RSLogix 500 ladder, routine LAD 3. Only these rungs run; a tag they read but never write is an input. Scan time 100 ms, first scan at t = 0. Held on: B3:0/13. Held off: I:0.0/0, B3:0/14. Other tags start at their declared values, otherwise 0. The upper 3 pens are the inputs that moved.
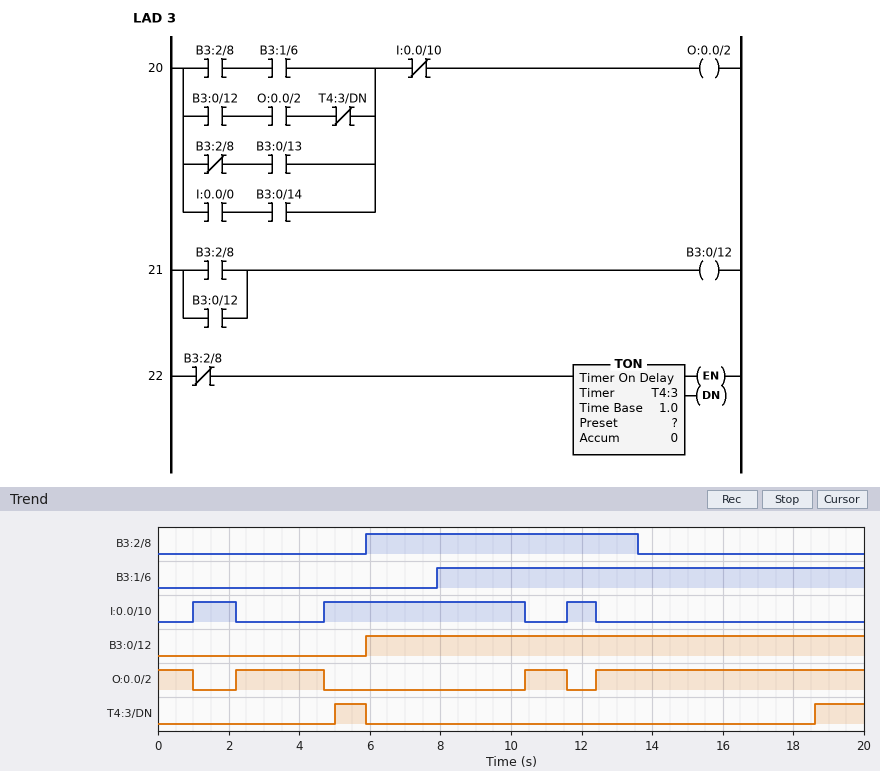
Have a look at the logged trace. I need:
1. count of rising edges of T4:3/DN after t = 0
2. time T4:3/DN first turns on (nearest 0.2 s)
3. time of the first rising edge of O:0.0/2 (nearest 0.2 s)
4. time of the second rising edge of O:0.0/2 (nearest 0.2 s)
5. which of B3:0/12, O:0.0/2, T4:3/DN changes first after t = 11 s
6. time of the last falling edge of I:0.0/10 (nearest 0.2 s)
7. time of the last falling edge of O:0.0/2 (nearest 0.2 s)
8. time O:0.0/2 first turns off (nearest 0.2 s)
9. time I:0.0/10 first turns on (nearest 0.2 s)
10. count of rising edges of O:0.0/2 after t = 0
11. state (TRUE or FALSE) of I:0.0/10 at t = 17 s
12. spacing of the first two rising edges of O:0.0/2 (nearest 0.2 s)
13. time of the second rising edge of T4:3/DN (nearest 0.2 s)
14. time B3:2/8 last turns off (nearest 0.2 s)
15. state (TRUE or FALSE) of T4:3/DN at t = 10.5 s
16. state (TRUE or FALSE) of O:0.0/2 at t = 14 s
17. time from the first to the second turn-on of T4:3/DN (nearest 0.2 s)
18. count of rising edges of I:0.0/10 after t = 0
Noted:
2
5.0 s
2.2 s
10.4 s
O:0.0/2
12.4 s
11.6 s
1.0 s
1.0 s
3
FALSE
8.2 s
18.6 s
13.6 s
FALSE
TRUE
13.6 s
3
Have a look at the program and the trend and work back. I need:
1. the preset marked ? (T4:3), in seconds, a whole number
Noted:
5 s
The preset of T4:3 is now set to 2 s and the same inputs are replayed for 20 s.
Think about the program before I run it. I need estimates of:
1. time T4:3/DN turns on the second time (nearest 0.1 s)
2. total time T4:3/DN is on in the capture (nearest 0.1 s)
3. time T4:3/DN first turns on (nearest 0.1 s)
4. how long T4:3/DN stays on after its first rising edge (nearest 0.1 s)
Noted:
15.6 s
8.3 s
2.0 s
3.9 s
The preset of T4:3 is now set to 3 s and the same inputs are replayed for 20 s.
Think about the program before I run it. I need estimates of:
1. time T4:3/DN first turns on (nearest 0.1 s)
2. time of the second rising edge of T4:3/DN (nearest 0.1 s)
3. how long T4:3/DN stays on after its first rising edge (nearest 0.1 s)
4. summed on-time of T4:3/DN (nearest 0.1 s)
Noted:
3.0 s
16.6 s
2.9 s
6.3 s
